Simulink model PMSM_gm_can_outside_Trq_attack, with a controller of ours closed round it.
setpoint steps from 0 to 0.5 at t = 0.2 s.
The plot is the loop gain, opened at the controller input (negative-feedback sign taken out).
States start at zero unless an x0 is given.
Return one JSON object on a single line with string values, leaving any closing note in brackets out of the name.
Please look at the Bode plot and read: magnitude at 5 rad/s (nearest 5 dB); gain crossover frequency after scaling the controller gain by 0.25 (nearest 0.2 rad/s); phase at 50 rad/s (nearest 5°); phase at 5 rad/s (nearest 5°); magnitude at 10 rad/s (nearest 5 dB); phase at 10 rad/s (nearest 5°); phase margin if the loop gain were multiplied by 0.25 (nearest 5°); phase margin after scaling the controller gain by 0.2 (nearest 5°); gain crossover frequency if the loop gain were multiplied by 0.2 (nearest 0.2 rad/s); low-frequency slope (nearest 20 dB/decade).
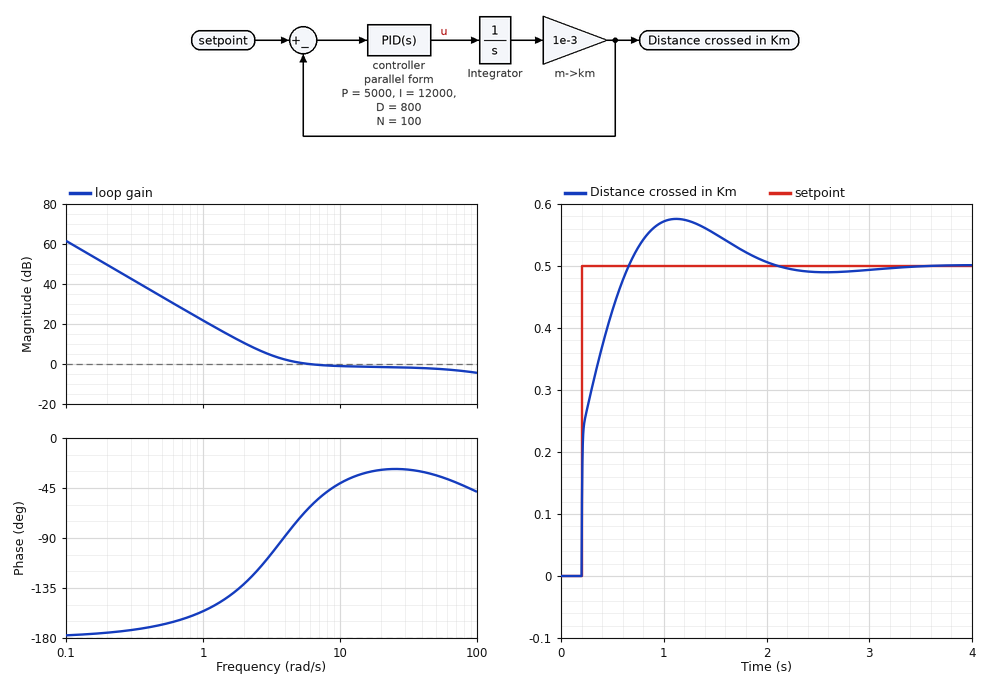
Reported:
{"magnitude at 5 rad/s": "0 dB", "gain crossover frequency after scaling the controller gain by 0.25": "1.8 rad/s", "phase at 50 rad/s": "-35°", "phase at 5 rad/s": "-75°", "magnitude at 10 rad/s": "0 dB", "phase at 10 rad/s": "-40°", "phase margin if the loop gain were multiplied by 0.25": "45°", "phase margin after scaling the controller gain by 0.2": "40°", "gain crossover frequency if the loop gain were multiplied by 0.2": "1.6 rad/s", "low-frequency slope": "-40 dB/decade"}
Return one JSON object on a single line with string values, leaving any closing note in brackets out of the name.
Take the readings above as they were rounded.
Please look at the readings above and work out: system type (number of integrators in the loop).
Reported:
{"system type": "2"}
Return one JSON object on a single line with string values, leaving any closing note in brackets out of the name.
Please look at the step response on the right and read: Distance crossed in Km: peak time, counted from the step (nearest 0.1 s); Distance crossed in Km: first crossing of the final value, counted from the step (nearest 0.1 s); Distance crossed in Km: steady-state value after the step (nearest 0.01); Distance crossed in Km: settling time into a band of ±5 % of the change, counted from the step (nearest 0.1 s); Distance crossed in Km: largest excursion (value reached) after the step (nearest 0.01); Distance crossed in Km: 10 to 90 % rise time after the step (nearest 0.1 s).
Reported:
{"Distance crossed in Km: peak time, counted from the step": "0.9 s", "Distance crossed in Km: first crossing of the final value, counted from the step": "0.5 s", "Distance crossed in Km: steady-state value after the step": "0.50", "Distance crossed in Km: settling time into a band of ±5 % of the change, counted from the step": "1.6 s", "Distance crossed in Km: largest excursion (value reached) after the step": "0.58", "Distance crossed in Km: 10 to 90 % rise time after the step": "0.3 s"}
